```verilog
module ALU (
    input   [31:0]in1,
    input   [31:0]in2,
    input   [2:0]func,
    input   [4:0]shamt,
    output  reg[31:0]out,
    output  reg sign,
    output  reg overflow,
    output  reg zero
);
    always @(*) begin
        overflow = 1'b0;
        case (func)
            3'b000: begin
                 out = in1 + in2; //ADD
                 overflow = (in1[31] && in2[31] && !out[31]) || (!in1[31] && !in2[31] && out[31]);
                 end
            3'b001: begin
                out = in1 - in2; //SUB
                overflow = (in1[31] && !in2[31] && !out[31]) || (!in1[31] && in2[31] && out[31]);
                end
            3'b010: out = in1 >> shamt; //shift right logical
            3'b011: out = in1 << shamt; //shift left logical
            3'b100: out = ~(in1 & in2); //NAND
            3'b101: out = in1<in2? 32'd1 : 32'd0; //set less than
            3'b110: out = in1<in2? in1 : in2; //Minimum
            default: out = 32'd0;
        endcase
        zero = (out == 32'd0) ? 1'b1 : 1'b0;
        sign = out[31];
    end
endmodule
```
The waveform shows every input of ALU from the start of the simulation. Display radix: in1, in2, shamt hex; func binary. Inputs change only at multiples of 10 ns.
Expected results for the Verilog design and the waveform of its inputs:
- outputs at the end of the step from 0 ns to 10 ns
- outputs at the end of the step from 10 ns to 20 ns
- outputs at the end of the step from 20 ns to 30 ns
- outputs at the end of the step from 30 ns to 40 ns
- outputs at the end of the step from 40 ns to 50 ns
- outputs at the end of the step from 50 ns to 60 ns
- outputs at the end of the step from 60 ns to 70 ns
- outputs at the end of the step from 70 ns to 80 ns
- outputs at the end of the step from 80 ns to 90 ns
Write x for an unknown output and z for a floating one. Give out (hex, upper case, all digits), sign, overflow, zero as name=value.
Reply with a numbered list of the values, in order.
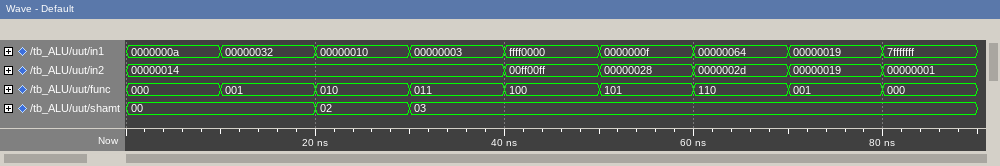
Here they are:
1. out=0000001E, sign=0, overflow=0, zero=0
2. out=0000001E, sign=0, overflow=0, zero=0
3. out=00000004, sign=0, overflow=0, zero=0
4. out=00000018, sign=0, overflow=0, zero=0
5. out=FF00FFFF, sign=1, overflow=0, zero=0
6. out=00000001, sign=0, overflow=0, zero=0
7. out=0000002D, sign=0, overflow=0, zero=0
8. out=00000000, sign=0, overflow=0, zero=1
9. out=80000000, sign=1, overflow=1, zero=0
